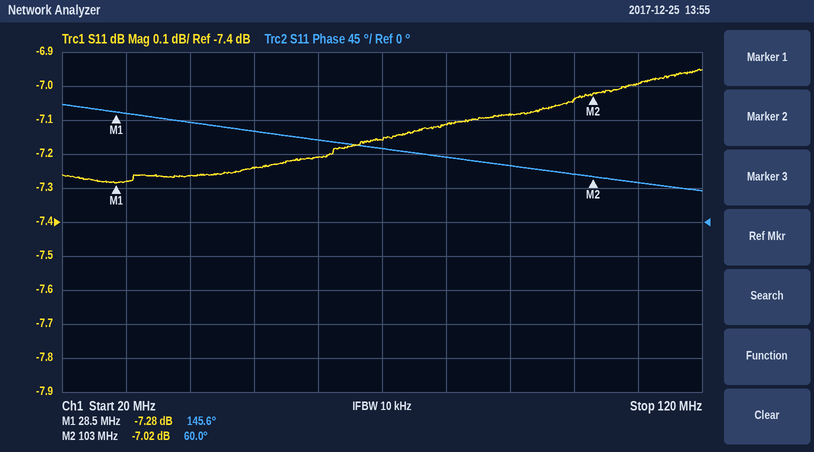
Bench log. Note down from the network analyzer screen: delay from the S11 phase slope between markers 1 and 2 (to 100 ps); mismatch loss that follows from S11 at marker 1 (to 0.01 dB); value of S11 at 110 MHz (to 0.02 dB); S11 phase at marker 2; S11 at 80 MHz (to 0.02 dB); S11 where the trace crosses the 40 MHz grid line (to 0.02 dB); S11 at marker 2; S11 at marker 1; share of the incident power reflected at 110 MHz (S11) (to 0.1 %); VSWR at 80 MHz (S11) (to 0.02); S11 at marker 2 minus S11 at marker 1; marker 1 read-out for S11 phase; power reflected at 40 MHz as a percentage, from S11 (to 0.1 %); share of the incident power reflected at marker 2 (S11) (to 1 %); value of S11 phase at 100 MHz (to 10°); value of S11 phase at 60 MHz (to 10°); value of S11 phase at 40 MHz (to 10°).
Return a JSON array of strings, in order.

["3.2 ns", "0.90 dB", "-7.00 dB", "60.0°", "-7.12 dB", "-7.26 dB", "-7.02 dB", "-7.28 dB", "20.0 %", "2.58", "0.26 dB", "145.6°", "18.8 %", "20 %", "60°", "110°", "130°"]
